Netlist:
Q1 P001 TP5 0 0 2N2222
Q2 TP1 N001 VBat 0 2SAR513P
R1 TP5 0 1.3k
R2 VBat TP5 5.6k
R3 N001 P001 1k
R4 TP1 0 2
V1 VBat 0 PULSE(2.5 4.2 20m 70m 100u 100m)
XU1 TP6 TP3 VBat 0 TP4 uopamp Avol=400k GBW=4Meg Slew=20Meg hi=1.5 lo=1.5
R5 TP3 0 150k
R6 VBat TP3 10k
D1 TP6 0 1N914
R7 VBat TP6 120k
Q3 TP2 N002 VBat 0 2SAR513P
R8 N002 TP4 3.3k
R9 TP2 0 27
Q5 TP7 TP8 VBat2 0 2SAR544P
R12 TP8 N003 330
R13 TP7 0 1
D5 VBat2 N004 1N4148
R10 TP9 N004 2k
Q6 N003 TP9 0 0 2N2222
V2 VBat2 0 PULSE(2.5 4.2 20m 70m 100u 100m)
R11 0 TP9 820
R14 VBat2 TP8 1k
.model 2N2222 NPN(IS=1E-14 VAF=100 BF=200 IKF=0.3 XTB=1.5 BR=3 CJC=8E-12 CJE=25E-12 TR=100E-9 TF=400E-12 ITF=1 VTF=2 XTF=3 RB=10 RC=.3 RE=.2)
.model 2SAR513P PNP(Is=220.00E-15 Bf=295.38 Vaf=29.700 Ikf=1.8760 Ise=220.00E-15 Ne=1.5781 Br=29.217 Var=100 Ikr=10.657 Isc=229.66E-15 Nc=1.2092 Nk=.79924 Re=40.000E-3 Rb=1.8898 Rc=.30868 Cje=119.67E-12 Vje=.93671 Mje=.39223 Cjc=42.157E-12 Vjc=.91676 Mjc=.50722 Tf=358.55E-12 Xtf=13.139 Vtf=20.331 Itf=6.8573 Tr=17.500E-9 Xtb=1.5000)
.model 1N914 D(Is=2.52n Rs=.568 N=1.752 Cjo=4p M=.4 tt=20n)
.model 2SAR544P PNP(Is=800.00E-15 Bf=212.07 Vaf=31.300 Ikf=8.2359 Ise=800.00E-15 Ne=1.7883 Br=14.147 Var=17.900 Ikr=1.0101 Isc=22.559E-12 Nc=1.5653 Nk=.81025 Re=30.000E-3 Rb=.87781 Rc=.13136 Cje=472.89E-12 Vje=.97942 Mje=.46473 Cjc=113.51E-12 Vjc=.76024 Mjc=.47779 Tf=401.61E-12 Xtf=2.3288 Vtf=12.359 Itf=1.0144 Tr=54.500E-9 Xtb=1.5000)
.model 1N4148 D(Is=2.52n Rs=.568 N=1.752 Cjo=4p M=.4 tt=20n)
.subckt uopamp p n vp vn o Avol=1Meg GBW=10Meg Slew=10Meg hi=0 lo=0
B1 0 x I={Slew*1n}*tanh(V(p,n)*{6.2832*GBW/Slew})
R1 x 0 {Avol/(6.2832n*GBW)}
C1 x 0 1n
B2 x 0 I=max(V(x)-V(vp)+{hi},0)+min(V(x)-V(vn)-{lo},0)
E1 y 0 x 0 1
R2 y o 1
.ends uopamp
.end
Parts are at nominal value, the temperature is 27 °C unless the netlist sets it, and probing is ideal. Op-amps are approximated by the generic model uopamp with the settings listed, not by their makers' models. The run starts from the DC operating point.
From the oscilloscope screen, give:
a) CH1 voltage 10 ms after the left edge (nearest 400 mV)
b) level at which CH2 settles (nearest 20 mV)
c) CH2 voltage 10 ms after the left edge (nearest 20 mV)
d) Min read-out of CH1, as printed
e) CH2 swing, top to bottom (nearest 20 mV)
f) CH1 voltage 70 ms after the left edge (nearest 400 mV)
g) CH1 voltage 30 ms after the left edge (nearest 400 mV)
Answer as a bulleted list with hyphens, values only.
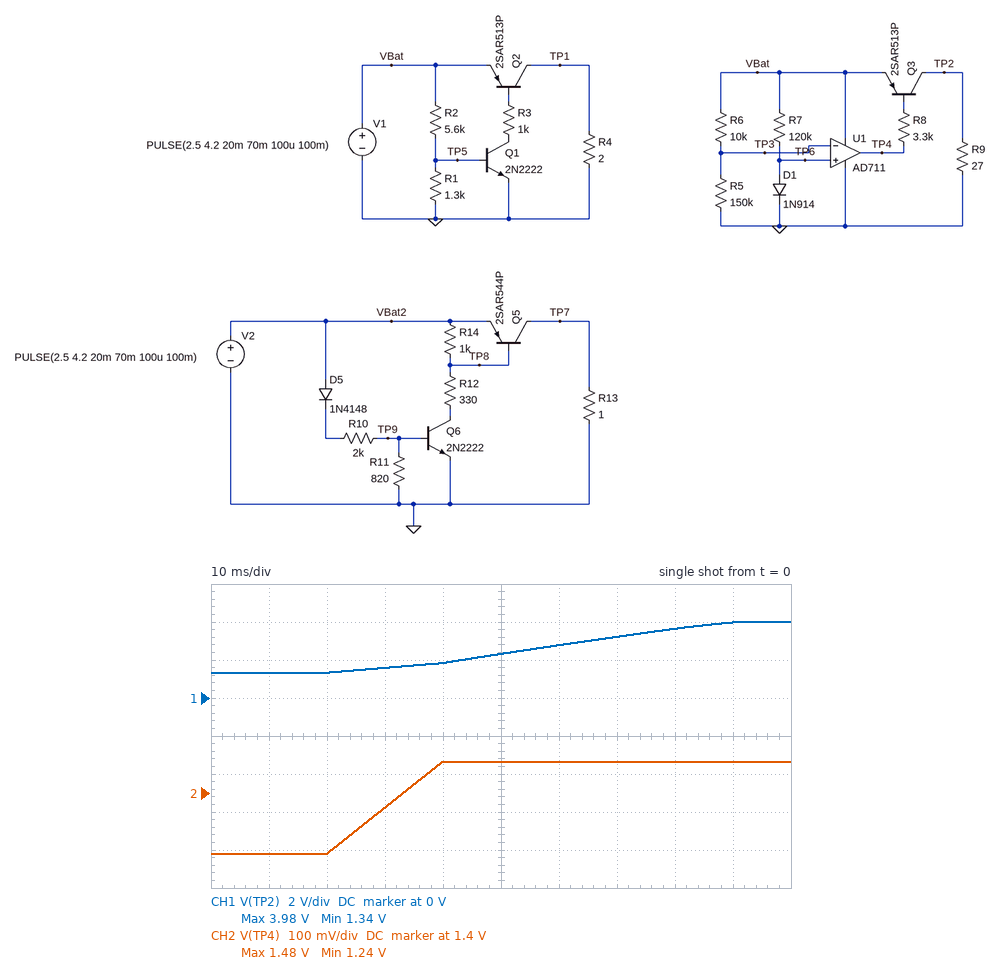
- 1.2 V
- 1.48 V
- 1.24 V
- 1.34 V
- 240 mV
- 3.2 V
- 1.6 V
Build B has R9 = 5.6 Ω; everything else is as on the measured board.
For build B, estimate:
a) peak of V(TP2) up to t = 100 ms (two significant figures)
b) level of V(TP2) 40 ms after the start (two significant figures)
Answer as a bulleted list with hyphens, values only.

- 930 mV
- 400 mV
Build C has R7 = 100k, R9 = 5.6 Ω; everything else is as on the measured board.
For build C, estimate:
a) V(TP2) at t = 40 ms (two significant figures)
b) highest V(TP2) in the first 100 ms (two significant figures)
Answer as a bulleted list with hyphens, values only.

- 400 mV
- 930 mV
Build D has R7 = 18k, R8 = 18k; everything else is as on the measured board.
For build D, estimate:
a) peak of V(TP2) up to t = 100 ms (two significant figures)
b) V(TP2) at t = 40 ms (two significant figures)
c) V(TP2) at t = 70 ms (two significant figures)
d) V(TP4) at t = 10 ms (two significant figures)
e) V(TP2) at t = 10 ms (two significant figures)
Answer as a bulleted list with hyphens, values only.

- 930 mV
- 390 mV
- 710 mV
- 1.2 V
- 280 mV
